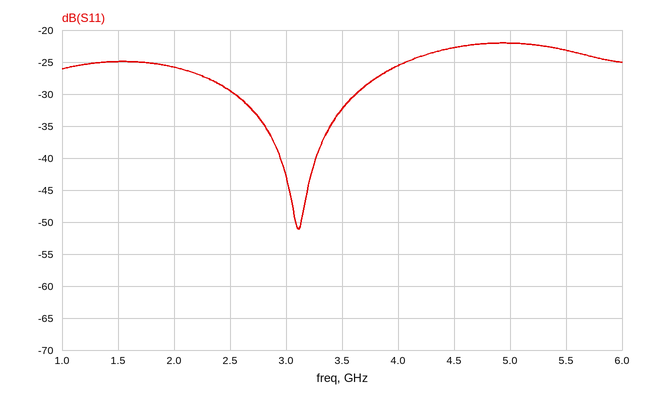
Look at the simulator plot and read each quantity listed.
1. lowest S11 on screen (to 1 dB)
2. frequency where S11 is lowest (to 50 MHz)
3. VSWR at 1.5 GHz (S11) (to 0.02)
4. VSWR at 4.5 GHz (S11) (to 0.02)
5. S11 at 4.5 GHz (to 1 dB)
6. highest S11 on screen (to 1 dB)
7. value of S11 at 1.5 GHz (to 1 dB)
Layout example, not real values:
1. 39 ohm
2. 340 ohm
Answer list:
1. -51 dB
2. 3.10 GHz
3. 1.12
4. 1.16
5. -23 dB
6. -22 dB
7. -25 dB
